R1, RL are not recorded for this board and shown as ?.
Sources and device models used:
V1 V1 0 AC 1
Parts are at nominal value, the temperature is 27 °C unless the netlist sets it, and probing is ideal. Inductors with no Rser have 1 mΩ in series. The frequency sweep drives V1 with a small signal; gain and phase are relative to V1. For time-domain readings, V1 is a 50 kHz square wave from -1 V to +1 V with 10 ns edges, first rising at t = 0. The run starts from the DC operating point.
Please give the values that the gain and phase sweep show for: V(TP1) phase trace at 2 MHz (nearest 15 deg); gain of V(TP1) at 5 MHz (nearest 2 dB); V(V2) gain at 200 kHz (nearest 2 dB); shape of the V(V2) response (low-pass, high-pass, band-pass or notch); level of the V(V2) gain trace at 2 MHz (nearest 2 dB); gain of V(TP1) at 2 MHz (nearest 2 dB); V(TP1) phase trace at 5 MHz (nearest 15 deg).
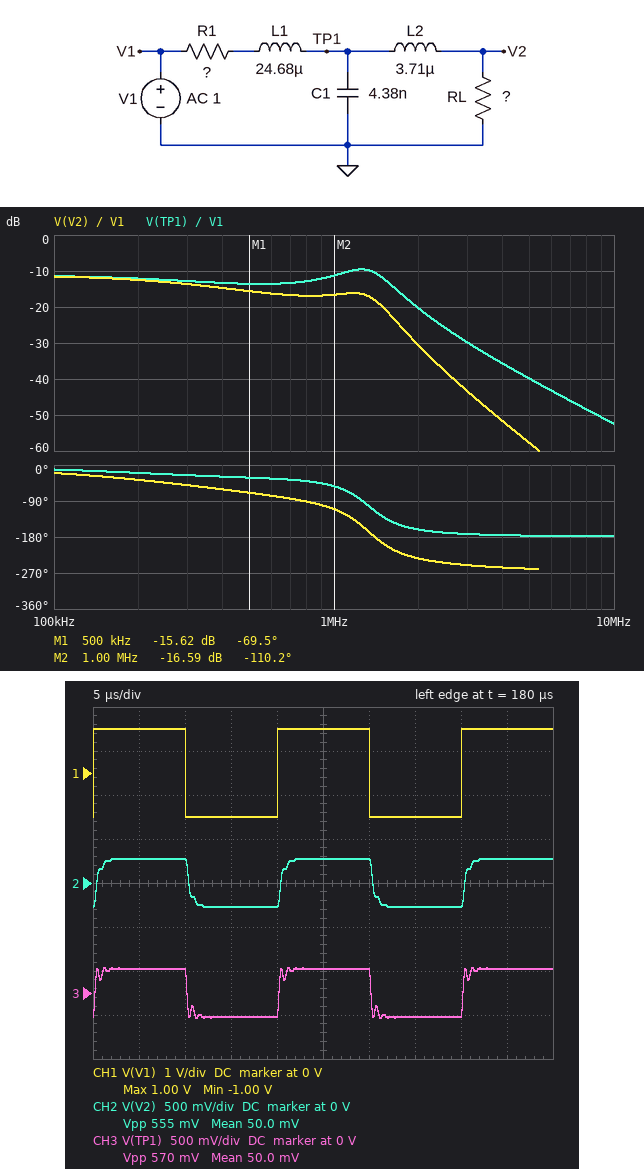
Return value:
-165 deg
-40 dB
-12 dB
low-pass
-30 dB
-20 dB
-180 deg
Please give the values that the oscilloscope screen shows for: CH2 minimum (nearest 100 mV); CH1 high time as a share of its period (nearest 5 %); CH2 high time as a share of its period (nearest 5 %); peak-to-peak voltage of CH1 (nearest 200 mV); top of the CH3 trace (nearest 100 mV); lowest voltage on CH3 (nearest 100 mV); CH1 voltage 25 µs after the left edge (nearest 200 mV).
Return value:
-300 mV
50 %
50 %
2.0 V
300 mV
-300 mV
1.0 V
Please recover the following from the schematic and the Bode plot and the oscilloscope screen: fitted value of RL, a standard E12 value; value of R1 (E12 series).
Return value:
15 Ω
39 Ω
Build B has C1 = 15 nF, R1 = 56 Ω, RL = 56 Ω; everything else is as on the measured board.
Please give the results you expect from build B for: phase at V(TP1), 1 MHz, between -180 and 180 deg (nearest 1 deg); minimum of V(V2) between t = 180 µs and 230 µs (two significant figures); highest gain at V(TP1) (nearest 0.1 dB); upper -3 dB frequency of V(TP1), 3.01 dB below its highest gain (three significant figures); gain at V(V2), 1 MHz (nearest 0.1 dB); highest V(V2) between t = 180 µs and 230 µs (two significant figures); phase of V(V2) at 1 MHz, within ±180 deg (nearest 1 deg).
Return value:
-148 deg
-530 mV
-6.0 dB
373 kHz
-23.5 dB
530 mV
-171 deg
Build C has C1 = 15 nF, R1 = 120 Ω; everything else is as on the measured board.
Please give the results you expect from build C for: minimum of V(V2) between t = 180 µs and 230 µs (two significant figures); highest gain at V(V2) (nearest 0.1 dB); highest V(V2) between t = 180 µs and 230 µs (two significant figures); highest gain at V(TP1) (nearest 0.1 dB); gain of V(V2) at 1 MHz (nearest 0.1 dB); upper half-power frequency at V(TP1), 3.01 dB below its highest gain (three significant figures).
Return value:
-140 mV
-18.8 dB
140 mV
-16.7 dB
-27.3 dB
871 kHz
